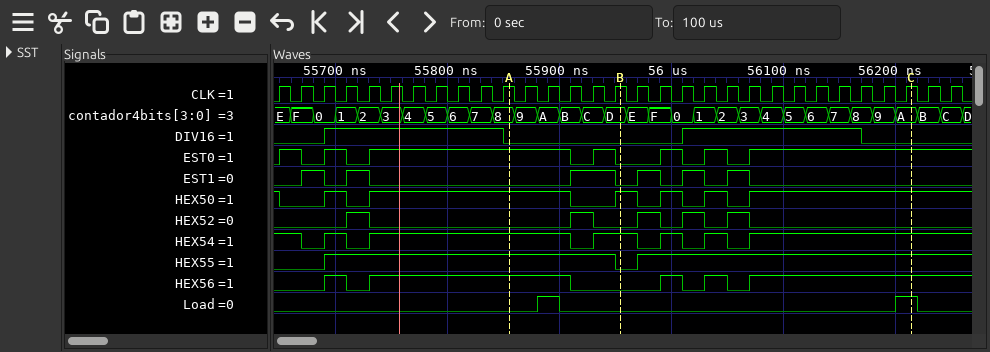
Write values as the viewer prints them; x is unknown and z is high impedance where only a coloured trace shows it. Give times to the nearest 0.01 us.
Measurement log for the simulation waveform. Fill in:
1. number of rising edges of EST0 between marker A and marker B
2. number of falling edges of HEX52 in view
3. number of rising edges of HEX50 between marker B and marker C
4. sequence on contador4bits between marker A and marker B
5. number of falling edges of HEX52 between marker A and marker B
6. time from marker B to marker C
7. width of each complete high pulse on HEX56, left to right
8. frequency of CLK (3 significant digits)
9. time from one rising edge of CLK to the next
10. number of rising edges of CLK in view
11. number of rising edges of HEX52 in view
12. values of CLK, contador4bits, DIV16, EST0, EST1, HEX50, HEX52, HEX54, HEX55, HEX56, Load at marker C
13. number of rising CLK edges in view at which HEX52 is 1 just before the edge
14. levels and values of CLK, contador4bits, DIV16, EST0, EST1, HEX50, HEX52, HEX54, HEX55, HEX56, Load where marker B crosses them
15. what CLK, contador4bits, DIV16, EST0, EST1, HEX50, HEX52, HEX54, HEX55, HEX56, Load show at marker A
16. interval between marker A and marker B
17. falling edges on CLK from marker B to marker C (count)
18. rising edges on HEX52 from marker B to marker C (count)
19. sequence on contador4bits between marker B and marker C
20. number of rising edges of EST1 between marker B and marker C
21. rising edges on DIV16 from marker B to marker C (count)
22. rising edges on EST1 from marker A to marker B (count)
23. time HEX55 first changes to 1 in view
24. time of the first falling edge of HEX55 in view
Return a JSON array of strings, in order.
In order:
["1", "5", "3", "8, 9, A, B, C, D", "1", "0.26 us", "0.02 us, 0.18 us, 0.02 us, 0.02 us", "50.0 MHz", "0.02 us", "31", "5", "CLK=1, contador4bits=A, DIV16=0, EST0=1, EST1=0, HEX50=1, HEX52=0, HEX54=1, HEX55=1, HEX56=1, Load=1", "5", "CLK=1, contador4bits=D, DIV16=0, EST0=0, EST1=0, HEX50=1, HEX52=0, HEX54=1, HEX55=0, HEX56=0, Load=0", "CLK=1, contador4bits=8, DIV16=0, EST0=1, EST1=0, HEX50=1, HEX52=0, HEX54=1, HEX55=1, HEX56=1, Load=0", "0.1 us", "13", "3", "D, E, F, 0, 1, 2, 3, 4, 5, 6, 7, 8, 9, A", "3", "1", "1", "55.69 us", "55.95 us"]
